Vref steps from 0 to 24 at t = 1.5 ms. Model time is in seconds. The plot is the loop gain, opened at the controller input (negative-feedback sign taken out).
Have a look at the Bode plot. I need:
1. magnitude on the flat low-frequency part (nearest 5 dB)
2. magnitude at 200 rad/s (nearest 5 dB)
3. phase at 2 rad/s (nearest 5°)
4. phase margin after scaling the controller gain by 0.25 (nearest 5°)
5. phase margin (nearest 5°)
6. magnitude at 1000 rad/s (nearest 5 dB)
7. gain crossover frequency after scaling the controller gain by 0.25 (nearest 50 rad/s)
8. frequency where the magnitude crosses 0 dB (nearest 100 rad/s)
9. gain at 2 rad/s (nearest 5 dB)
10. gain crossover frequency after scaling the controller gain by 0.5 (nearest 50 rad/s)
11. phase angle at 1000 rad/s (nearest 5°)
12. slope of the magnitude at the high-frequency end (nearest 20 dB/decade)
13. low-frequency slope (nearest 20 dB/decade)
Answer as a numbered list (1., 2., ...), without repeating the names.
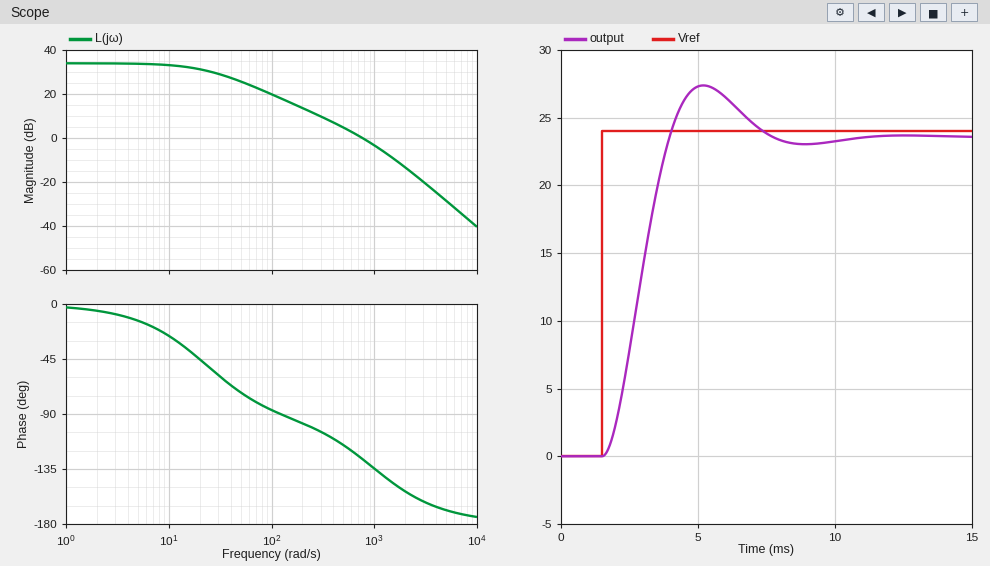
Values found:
1. 35 dB
2. 15 dB
3. -5°
4. 80°
5. 55°
6. -5 dB
7. 250 rad/s
8. 800 rad/s
9. 35 dB
10. 450 rad/s
11. -135°
12. -40 dB/decade
13. 0 dB/decade
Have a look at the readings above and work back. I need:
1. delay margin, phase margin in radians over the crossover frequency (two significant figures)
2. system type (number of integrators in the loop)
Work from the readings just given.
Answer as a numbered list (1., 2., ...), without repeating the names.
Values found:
1. 0.0012 s
2. 0
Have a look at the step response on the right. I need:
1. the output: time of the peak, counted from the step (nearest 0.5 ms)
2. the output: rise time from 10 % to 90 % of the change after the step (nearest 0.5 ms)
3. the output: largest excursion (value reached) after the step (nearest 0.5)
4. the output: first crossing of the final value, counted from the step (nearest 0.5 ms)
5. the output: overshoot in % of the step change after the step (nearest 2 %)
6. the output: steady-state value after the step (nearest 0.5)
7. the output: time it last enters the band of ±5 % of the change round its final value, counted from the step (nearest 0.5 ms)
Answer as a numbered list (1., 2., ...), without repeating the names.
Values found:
1. 3.5 ms
2. 1.5 ms
3. 27.5
4. 2.5 ms
5. 16 %
6. 23.5
7. 5.5 ms
